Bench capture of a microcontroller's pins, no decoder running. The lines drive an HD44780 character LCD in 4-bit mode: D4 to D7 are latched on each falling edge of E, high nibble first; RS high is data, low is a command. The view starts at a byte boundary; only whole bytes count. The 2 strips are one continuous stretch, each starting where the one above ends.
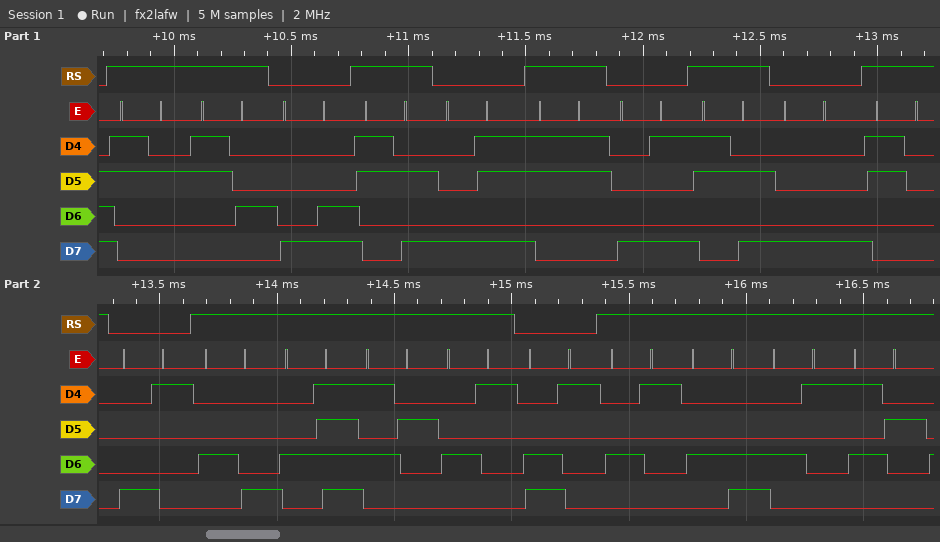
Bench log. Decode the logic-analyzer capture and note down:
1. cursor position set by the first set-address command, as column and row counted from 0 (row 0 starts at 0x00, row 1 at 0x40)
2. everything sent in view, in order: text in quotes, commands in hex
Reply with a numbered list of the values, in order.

1. column 12, row 0
2. "24" 0x8C ":" 0x8B "3" 0x89 ":" 0x88 "0" 0x81 "HORA" 0xC1 "ALAR"
